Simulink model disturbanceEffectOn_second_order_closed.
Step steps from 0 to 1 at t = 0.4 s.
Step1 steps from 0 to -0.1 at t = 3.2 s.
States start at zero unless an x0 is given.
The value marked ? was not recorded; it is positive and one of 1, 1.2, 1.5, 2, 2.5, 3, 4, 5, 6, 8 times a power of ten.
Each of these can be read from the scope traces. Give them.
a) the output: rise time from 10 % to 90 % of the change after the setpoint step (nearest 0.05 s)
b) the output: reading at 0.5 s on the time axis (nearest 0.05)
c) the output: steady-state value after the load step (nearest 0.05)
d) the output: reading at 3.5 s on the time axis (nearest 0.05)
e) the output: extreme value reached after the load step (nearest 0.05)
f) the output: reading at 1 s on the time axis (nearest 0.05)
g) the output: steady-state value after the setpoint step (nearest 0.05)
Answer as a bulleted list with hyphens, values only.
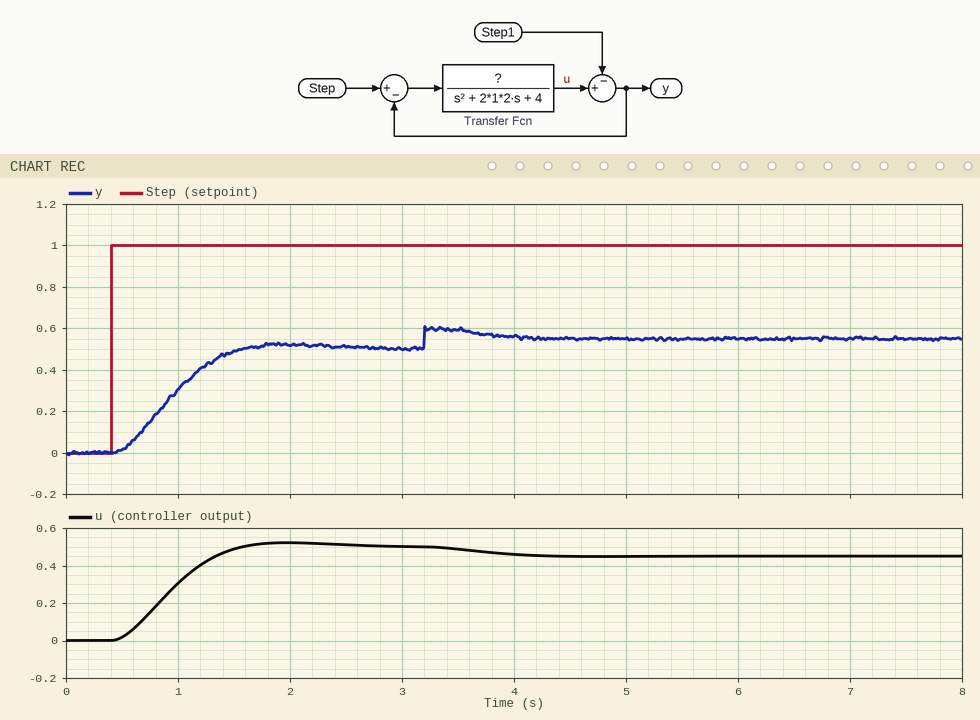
- 0.75 s
- 0.00
- 0.55
- 0.60
- 0.60
- 0.30
- 0.50
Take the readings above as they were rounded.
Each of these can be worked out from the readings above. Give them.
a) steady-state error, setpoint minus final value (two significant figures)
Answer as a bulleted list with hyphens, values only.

- 0.50
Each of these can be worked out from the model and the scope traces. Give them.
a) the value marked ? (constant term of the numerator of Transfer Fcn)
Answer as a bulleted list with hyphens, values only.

- 4
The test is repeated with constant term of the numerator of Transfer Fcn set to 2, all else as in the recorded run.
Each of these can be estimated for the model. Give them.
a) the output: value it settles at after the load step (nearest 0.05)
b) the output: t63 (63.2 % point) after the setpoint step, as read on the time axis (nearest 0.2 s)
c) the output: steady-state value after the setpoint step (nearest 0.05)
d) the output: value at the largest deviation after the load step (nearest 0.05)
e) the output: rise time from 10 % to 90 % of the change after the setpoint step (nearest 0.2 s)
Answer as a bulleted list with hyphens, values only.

- 0.40
- 1.2 s
- 0.35
- 0.45
- 1.0 s
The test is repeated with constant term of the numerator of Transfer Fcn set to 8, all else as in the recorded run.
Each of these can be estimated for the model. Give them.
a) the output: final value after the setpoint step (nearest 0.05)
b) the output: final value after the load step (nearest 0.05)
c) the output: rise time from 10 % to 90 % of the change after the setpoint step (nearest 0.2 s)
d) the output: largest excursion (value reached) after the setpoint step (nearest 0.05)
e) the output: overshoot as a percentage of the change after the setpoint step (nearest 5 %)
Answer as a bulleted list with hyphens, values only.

- 0.65
- 0.70
- 0.6 s
- 0.75
- 10 %
